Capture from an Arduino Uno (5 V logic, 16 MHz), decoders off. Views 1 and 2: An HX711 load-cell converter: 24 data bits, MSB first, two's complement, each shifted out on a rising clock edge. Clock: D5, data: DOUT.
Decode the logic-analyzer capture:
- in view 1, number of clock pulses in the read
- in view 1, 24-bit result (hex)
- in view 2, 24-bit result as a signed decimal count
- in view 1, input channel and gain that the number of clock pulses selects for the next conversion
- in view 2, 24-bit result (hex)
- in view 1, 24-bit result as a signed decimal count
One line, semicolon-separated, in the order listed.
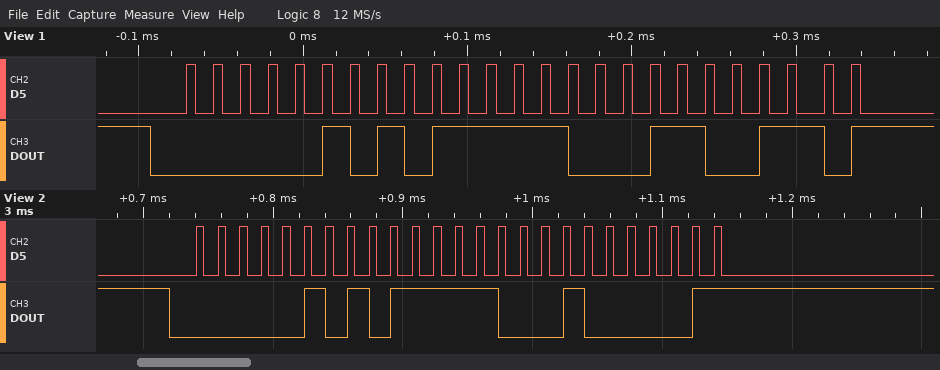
25; 0x057C66; 359489; channel A, gain 128; 0x057C41; 359526
